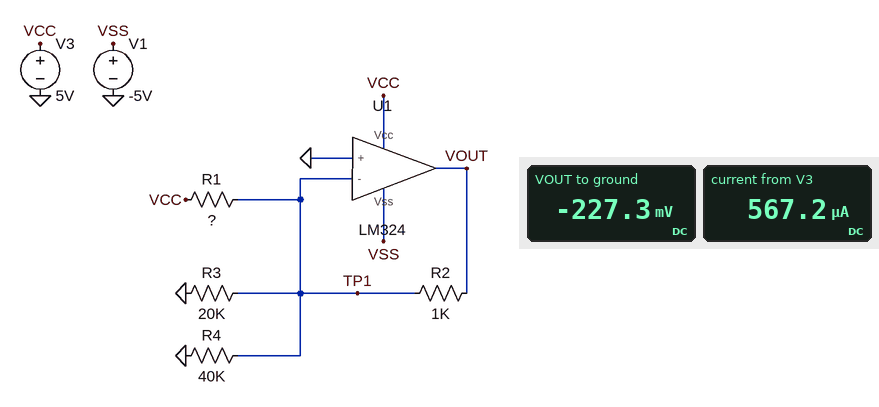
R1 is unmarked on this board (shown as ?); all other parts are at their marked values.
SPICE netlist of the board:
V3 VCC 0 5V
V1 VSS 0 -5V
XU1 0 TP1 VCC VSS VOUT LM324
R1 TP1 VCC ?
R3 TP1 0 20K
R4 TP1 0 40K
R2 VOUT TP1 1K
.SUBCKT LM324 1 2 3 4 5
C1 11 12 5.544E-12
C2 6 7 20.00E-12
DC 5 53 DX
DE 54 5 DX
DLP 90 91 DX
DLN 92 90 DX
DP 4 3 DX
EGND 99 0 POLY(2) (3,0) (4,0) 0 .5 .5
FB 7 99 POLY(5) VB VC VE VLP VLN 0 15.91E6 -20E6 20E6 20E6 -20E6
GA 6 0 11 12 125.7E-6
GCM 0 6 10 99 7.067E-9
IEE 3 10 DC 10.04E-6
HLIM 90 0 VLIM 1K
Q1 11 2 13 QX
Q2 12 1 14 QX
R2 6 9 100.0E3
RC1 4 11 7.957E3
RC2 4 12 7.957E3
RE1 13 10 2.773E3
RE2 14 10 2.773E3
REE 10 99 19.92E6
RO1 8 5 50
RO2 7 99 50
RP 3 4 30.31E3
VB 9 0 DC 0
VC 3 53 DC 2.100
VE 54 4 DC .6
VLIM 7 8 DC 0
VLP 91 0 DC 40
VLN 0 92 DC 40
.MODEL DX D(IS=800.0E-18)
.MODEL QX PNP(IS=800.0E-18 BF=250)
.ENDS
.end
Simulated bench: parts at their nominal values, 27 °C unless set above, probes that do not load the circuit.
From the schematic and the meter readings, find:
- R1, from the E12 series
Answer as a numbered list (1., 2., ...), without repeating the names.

1. 22 kΩ
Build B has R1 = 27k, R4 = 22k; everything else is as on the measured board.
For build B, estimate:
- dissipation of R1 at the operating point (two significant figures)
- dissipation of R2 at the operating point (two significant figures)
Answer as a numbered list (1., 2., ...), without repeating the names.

1. 930 µW
2. 34 µW
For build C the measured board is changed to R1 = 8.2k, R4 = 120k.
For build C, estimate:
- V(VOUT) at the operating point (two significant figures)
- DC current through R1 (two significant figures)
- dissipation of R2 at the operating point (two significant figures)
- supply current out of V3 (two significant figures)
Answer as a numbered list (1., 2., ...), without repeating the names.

1. -610 mV
2. 610 µA
3. 370 µW
4. 950 µA
